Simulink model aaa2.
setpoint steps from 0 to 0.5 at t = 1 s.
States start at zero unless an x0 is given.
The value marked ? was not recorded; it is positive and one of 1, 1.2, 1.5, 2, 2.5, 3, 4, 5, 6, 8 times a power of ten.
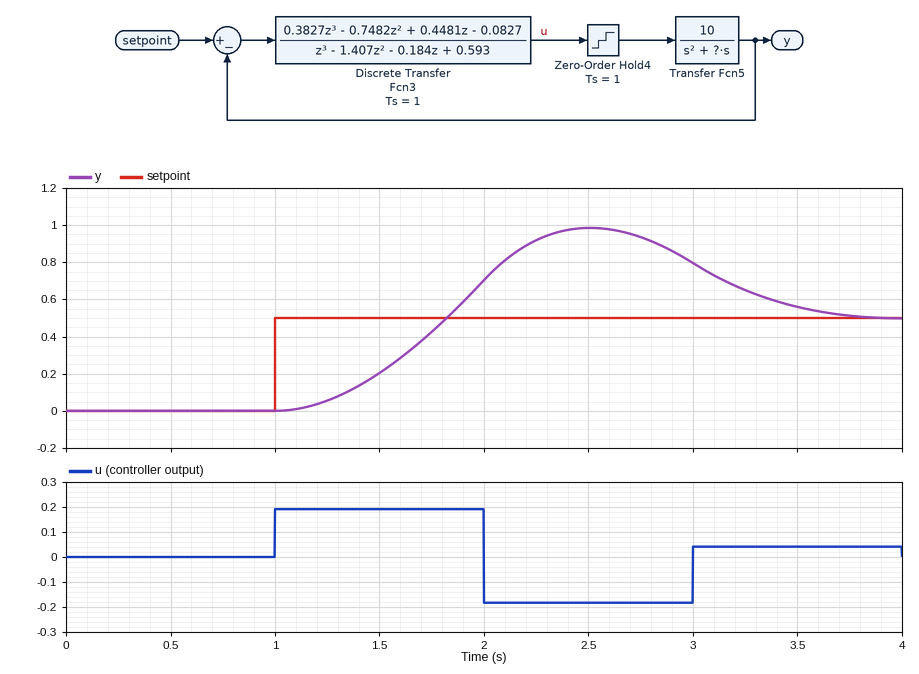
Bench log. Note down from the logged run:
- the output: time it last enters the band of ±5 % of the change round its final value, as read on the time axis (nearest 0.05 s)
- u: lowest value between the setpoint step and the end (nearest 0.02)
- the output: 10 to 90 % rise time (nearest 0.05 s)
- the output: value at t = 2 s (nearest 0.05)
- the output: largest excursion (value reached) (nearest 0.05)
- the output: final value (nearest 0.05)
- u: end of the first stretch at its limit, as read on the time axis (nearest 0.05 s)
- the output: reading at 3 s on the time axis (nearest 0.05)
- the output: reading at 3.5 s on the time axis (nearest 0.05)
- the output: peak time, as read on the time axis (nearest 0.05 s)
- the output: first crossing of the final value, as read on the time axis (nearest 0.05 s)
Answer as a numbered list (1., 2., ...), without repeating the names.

1. 3.65 s
2. -0.18
3. 0.55 s
4. 0.70
5. 1.00
6. 0.50
7. 2.00 s
8. 0.80
9. 0.55
10. 2.50 s
11. 1.80 s
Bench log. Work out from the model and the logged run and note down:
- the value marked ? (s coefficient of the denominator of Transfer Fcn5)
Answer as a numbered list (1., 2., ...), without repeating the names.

1. 1
